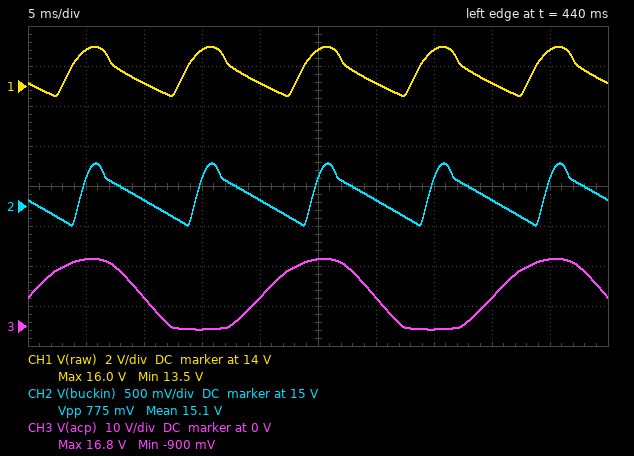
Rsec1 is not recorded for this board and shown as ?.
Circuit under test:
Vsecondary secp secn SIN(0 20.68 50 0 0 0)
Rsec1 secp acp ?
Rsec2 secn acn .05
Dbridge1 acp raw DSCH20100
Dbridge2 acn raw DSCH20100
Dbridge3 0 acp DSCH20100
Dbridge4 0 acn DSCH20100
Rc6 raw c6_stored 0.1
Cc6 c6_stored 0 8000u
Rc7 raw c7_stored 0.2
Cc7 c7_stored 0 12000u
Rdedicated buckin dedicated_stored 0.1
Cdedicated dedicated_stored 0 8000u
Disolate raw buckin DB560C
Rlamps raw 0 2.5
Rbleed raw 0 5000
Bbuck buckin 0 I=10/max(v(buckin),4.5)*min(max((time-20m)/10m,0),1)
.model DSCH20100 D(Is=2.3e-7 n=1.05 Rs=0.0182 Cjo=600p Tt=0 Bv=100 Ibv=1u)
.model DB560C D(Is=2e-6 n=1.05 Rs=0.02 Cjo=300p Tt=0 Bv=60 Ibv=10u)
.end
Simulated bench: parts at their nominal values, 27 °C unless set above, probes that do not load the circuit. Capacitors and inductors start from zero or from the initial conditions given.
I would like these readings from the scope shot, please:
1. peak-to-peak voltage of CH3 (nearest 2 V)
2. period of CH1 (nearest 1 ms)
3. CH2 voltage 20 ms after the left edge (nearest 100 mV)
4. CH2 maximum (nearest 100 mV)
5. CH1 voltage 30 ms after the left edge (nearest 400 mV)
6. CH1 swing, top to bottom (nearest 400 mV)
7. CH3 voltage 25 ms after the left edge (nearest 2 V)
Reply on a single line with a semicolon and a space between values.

18 V; 10 ms; 15.1 V; 15.5 V; 14.0 V; 2.4 V; 16 V
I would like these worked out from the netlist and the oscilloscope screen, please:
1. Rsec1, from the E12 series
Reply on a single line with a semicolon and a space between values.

0.1 Ω
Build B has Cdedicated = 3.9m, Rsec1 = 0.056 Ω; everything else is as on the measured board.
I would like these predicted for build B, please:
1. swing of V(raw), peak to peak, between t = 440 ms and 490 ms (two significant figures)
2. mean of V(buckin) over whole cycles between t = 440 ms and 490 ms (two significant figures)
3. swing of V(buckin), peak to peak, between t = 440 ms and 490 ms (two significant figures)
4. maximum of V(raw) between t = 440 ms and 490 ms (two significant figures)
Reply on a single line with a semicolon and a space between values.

2.7 V; 16 V; 1.3 V; 17 V
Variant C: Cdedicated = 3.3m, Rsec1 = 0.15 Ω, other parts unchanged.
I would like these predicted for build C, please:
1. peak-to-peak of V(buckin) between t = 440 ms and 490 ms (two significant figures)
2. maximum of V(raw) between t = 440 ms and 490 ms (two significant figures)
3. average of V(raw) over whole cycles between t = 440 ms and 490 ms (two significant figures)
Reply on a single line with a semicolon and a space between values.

1.5 V; 15 V; 14 V
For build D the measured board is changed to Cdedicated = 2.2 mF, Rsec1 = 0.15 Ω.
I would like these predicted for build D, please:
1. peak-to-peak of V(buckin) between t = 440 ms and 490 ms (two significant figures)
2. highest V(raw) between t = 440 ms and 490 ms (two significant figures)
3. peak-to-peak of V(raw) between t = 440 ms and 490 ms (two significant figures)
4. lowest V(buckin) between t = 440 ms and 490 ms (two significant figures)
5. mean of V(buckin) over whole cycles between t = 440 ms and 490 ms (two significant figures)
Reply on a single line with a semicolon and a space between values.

2.1 V; 15 V; 2.4 V; 13 V; 14 V
